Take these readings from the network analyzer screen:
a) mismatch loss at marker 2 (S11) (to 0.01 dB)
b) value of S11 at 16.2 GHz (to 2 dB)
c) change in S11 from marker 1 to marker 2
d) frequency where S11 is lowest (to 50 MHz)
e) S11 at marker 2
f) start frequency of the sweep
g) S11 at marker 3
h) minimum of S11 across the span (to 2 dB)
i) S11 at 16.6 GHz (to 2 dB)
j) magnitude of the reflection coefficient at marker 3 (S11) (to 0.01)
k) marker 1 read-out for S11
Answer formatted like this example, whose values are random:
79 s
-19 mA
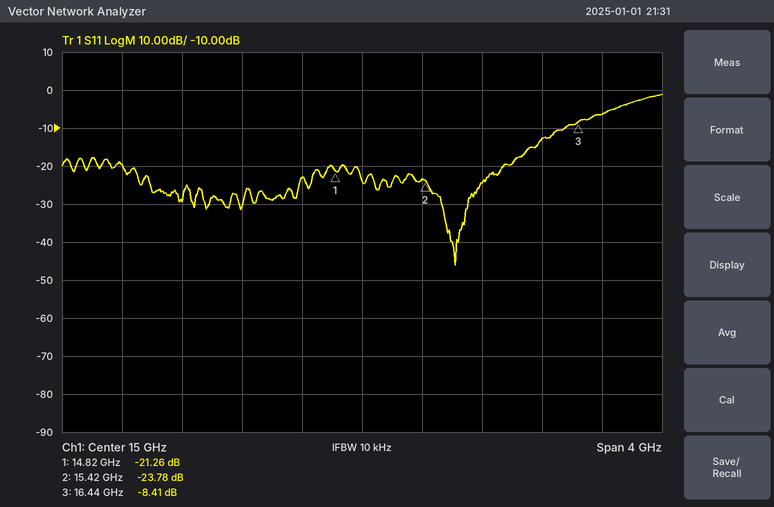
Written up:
0.02 dB
-12 dB
-2.52 dB
15.60 GHz
-23.78 dB
13 GHz
-8.41 dB
-46 dB
-6 dB
0.38
-21.26 dB
